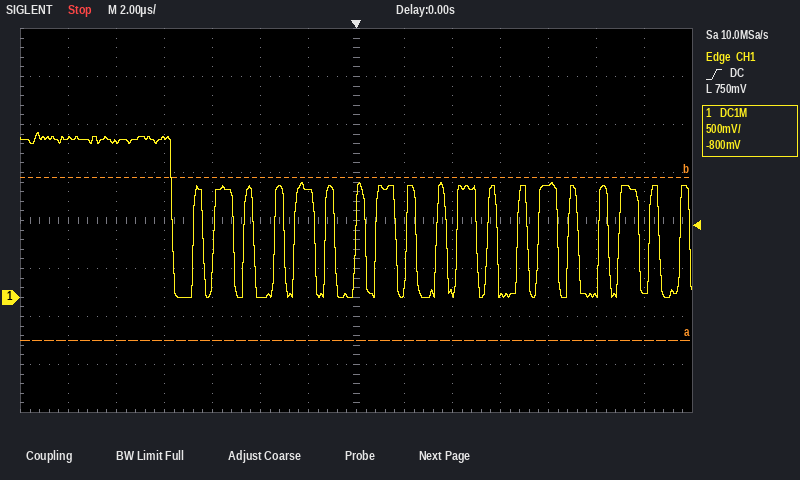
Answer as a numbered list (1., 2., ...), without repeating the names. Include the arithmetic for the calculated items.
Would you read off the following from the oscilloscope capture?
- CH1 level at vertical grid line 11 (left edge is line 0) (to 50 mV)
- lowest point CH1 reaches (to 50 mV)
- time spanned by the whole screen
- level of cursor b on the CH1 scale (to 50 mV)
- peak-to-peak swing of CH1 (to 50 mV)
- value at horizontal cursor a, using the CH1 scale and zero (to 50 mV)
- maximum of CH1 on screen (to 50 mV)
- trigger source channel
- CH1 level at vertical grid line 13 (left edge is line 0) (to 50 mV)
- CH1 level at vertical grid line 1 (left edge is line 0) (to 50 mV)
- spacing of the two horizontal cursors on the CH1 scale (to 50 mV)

1. 1.15 V
2. 0 mV
3. 28 µs
4. 1.25 V
5. 1.70 V − (0 mV) = 1.70 V
6. -450 mV
7. 1.70 V
8. CH1
9. 50 mV
10. 1.65 V
11. 1.70 V
